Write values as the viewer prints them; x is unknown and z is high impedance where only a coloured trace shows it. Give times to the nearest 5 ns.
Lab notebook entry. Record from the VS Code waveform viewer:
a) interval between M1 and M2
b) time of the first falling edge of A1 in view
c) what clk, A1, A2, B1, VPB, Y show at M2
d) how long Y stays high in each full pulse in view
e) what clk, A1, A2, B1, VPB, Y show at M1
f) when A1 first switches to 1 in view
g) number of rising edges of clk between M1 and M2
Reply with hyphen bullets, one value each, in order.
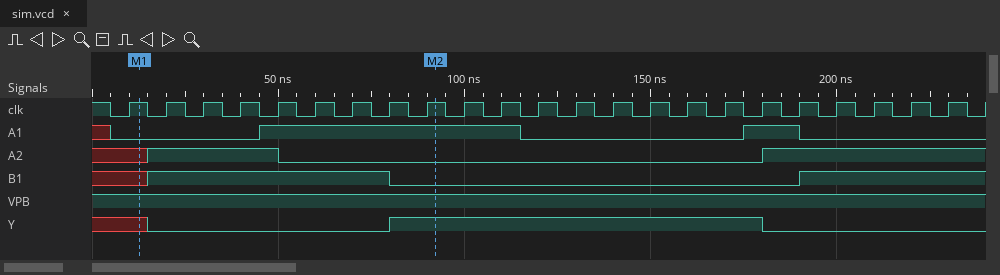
- 80 ns
- 115 ns
- clk=1, A1=1, A2=0, B1=0, VPB=1, Y=1
- 100 ns
- clk=1, A1=0, A2=x, B1=x, VPB=1, Y=x
- 45 ns
- 8
